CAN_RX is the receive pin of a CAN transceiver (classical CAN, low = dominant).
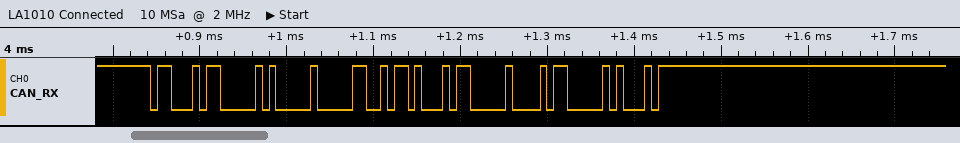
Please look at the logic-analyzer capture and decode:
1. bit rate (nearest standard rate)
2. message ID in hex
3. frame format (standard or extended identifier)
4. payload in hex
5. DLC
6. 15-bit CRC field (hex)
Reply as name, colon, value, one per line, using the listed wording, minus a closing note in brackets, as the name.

bit rate: 125 kbit/s
message ID in hex: 0x62C
frame format: standard
payload in hex: 00 96 8B 00
DLC: 4
15-bit CRC field: 0x2C08
